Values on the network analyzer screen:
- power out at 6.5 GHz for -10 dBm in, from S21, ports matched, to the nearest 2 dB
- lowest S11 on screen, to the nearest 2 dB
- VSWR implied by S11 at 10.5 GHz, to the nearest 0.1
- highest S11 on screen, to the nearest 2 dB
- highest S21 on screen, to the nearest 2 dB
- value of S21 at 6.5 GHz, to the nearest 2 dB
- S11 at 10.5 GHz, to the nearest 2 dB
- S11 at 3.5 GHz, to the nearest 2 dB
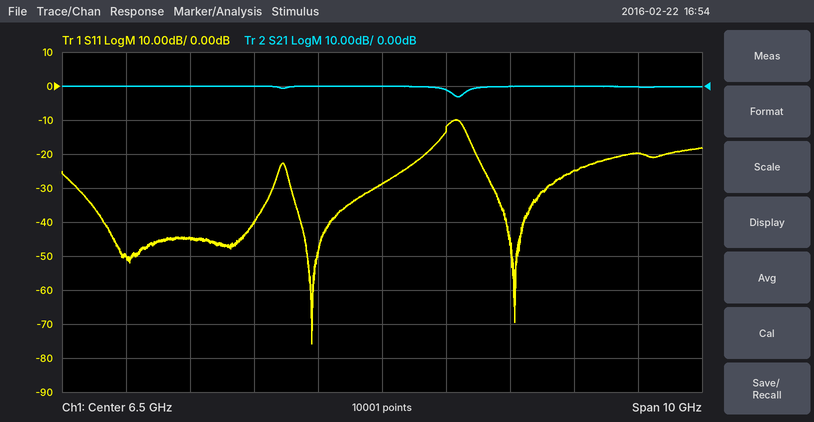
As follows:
-10 dBm
-76 dB
1.2
-10 dB
0 dB
0 dB
-20 dB
-44 dB
